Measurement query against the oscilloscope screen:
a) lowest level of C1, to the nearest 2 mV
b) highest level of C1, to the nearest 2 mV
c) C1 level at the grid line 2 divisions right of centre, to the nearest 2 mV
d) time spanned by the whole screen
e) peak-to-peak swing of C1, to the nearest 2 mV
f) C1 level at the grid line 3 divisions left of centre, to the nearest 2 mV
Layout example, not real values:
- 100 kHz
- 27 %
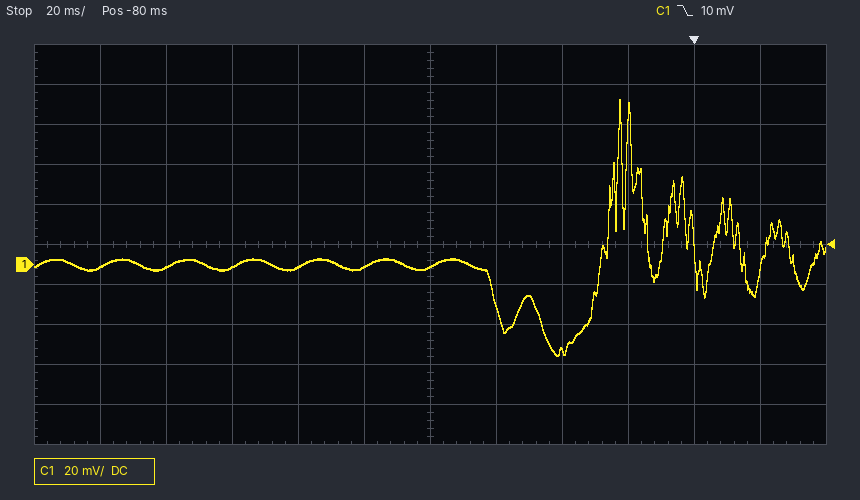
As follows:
- -46 mV
- 82 mV
- -44 mV
- 240 ms
- 128 mV
- -2 mV
